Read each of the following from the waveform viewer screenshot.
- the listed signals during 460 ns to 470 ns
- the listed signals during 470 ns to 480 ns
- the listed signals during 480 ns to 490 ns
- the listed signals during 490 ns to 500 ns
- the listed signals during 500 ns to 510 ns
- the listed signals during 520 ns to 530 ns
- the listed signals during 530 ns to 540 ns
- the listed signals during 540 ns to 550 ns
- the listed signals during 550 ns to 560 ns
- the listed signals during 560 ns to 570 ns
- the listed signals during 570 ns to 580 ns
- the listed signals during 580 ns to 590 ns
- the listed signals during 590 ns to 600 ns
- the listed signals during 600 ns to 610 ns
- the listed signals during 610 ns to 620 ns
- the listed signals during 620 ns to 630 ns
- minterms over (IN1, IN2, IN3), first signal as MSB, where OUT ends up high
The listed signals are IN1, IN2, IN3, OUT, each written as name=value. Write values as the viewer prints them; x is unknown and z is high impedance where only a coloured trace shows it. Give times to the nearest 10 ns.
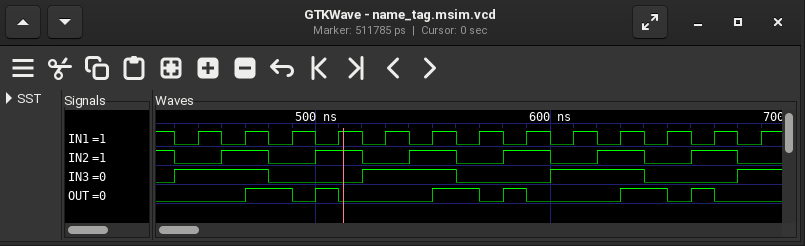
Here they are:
IN1=0, IN2=1, IN3=1, OUT=0
IN1=1, IN2=1, IN3=1, OUT=1
IN1=0, IN2=0, IN3=0, OUT=1
IN1=1, IN2=0, IN3=0, OUT=0
IN1=0, IN2=1, IN3=0, OUT=1
IN1=0, IN2=0, IN3=1, OUT=0
IN1=1, IN2=0, IN3=1, OUT=0
IN1=0, IN2=1, IN3=1, OUT=0
IN1=1, IN2=1, IN3=1, OUT=1
IN1=0, IN2=0, IN3=0, OUT=1
IN1=1, IN2=0, IN3=0, OUT=0
IN1=0, IN2=1, IN3=0, OUT=1
IN1=1, IN2=1, IN3=0, OUT=0
IN1=0, IN2=0, IN3=1, OUT=0
IN1=1, IN2=0, IN3=1, OUT=0
IN1=0, IN2=1, IN3=1, OUT=0
0, 2, 7
